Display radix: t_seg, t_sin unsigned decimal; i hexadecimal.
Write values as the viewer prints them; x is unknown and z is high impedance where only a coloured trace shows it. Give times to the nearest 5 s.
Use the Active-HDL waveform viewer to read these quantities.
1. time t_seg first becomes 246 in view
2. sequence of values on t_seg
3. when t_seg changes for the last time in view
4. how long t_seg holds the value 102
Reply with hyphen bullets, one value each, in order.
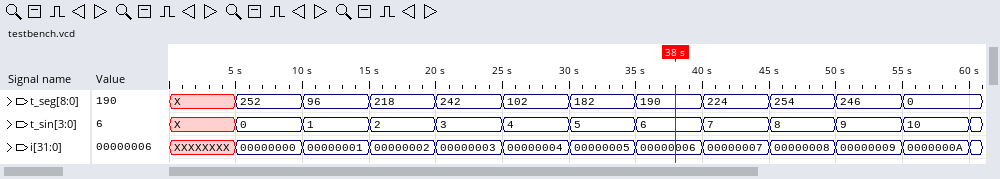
- 50 s
- X, 252, 96, 218, 242, 102, 182, 190, 224, 254, 246, 0
- 55 s
- 5 s
